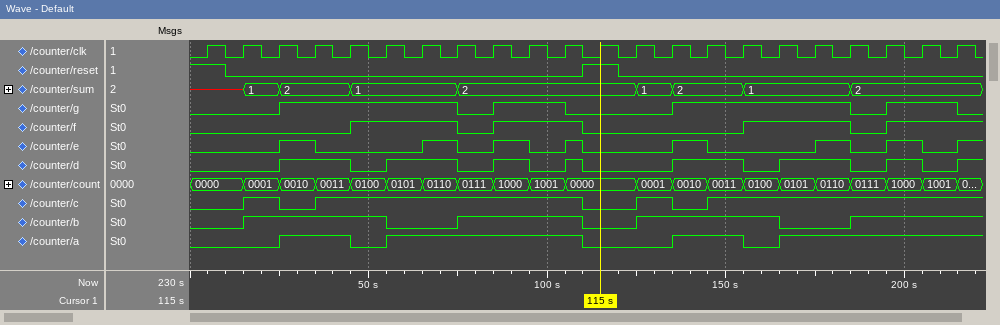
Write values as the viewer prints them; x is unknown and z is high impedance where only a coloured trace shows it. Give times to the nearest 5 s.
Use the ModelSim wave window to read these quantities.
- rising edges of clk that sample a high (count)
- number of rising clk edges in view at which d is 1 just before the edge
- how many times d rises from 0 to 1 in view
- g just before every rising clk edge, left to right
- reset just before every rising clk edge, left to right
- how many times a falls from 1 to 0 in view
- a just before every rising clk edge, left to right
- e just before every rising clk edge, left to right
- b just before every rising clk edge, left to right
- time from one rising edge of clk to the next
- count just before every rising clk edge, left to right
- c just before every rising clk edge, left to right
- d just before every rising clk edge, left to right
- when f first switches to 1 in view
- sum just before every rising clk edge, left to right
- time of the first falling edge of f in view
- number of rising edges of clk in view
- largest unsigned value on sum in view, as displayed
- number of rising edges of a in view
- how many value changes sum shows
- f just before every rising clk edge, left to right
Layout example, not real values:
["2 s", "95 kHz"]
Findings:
["14", "10", "8", "0 0 0 1 1 1 1 1 0 1 1 0 0 0 1 1 1 1 1 0 1 1", "1 0 0 0 0 0 0 0 0 0 0 1 0 0 0 0 0 0 0 0 0 0", "3", "0 0 0 1 1 0 1 1 1 1 1 0 0 0 1 1 0 1 1 1 1 1", "0 0 0 1 0 0 0 1 0 1 0 0 0 0 1 0 0 0 1 0 1 0", "0 0 1 1 1 1 0 0 1 1 1 0 0 1 1 1 1 0 0 1 1 1", "10 s", "0000, 0000, 0001, 0010, 0011, 0100, 0101, 0110, 0111, 1000, 1001, 0000, 0000, 0001, 0010, 0011, 0100, 0101, 0110, 0111, 1000, 1001", "0 0 1 0 1 1 1 1 1 1 1 0 0 1 0 1 1 1 1 1 1 1", "0 0 0 1 1 0 1 1 0 1 0 0 0 0 1 1 0 1 1 0 1 0", "45 s", "x, x, 1, 2, 2, 1, 1, 1, 2, 2, 2, 2, 2, 1, 2, 2, 1, 1, 1, 2, 2, 2", "75 s", "22", "2", "4", "8", "0 0 0 0 0 1 1 1 0 1 1 0 0 0 0 0 1 1 1 0 1 1"]
